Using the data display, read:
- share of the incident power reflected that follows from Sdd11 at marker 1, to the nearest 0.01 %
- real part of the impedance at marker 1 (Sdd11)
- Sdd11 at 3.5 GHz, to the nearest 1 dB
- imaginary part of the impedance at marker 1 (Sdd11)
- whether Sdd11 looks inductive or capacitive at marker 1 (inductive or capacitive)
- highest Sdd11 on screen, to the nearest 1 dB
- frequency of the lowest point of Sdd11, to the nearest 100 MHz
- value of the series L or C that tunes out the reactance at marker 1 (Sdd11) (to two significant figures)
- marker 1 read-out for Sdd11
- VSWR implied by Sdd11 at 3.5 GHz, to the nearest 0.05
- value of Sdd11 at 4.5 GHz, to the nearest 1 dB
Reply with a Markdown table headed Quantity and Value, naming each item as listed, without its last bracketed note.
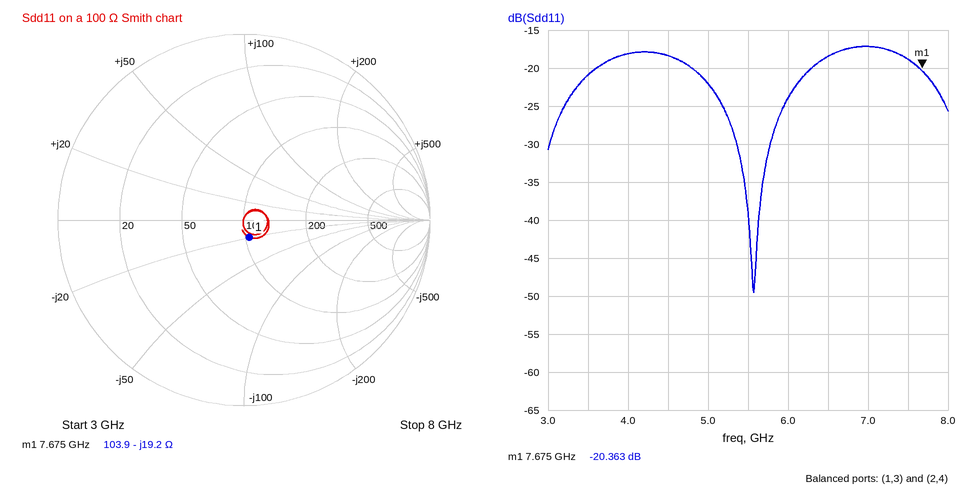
| Quantity | Value |
|---|---|
| share of the incident power reflected that follows from Sdd11 at marker 1, to the nearest 0.01 % | 0.92 % |
| real part of the impedance at marker 1 | 103.9 Ω |
| Sdd11 at 3.5 GHz, to the nearest 1 dB | -21 dB |
| imaginary part of the impedance at marker 1 | -19.2 Ω |
| whether Sdd11 looks inductive or capacitive at marker 1 | capacitive |
| highest Sdd11 on screen, to the nearest 1 dB | -17 dB |
| frequency of the lowest point of Sdd11, to the nearest 100 MHz | 5.6 GHz |
| value of the series L or C that tunes out the reactance at marker 1 (Sdd11) | 400 pH |
| marker 1 read-out for Sdd11 | -20.363 dB |
| VSWR implied by Sdd11 at 3.5 GHz, to the nearest 0.05 | 1.20 |
| value of Sdd11 at 4.5 GHz, to the nearest 1 dB | -18 dB |
